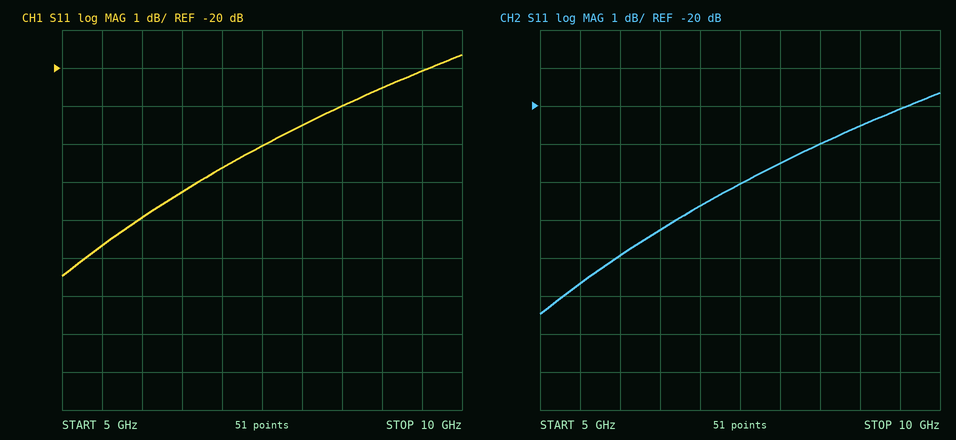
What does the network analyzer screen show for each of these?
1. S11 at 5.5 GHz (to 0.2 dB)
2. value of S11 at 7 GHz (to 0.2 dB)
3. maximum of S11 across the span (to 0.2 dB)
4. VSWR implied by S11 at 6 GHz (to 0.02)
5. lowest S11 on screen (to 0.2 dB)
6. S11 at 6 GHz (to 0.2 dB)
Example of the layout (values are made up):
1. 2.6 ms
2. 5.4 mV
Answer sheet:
1. -24.6 dB
2. -22.6 dB
3. -19.6 dB
4. 1.14
5. -25.4 dB
6. -24.0 dB
